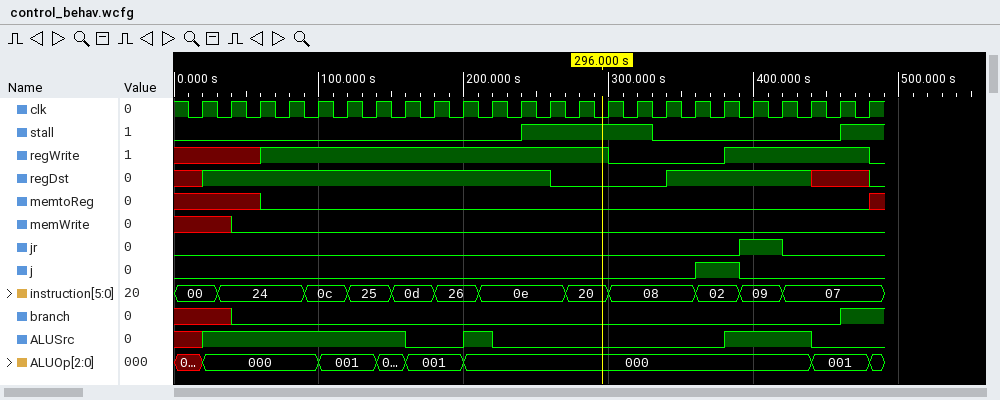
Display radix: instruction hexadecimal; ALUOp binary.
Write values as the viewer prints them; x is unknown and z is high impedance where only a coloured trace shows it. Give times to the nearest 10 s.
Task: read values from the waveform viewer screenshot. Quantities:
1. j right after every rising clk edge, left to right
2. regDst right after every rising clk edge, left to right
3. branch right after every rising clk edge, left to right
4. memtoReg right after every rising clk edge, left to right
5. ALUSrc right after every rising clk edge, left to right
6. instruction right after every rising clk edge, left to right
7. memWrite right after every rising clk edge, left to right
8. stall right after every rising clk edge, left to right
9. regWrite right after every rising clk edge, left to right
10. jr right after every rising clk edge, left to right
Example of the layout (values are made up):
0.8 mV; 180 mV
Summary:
0 0 0 0 0 0 0 0 0 0 0 0 0 0 0 0 0 1 1 0 0 0 0 0; 1 1 1 1 1 1 1 1 1 1 1 1 0 0 0 0 1 1 1 1 1 x x 0; x 0 0 0 0 0 0 0 0 0 0 0 0 0 0 0 0 0 0 0 0 0 1 1; x x 0 0 0 0 0 0 0 0 0 0 0 0 0 0 0 0 0 0 0 0 0 x; 1 1 1 1 1 1 1 0 0 1 0 0 0 0 0 0 0 0 1 1 1 0 0 0; 00, 24, 24, 24, 0c, 25, 25, 0d, 26, 26, 0e, 0e, 0e, 20, 08, 08, 08, 02, 02, 09, 07, 07, 07, 07; x 0 0 0 0 0 0 0 0 0 0 0 0 0 0 0 0 0 0 0 0 0 0 0; 0 0 0 0 0 0 0 0 0 0 0 1 1 1 1 1 0 0 0 0 0 0 1 1; x x 1 1 1 1 1 1 1 1 1 1 1 1 0 0 0 0 1 1 1 1 1 0; 0 0 0 0 0 0 0 0 0 0 0 0 0 0 0 0 0 0 0 1 0 0 0 0
